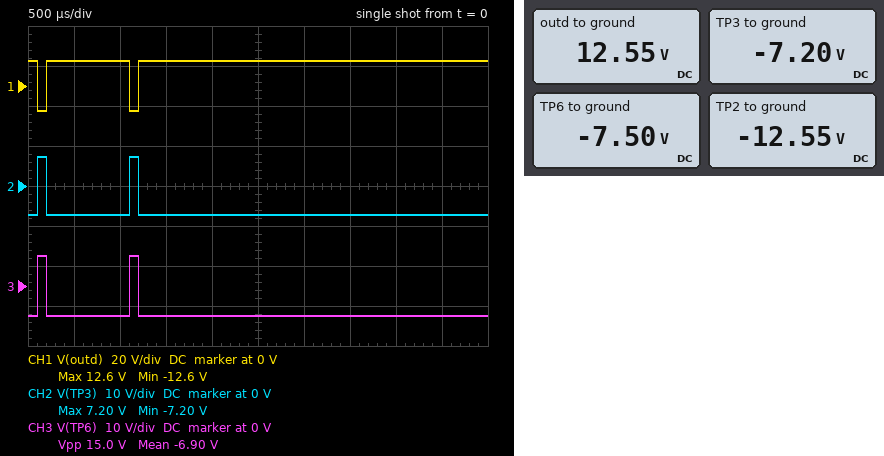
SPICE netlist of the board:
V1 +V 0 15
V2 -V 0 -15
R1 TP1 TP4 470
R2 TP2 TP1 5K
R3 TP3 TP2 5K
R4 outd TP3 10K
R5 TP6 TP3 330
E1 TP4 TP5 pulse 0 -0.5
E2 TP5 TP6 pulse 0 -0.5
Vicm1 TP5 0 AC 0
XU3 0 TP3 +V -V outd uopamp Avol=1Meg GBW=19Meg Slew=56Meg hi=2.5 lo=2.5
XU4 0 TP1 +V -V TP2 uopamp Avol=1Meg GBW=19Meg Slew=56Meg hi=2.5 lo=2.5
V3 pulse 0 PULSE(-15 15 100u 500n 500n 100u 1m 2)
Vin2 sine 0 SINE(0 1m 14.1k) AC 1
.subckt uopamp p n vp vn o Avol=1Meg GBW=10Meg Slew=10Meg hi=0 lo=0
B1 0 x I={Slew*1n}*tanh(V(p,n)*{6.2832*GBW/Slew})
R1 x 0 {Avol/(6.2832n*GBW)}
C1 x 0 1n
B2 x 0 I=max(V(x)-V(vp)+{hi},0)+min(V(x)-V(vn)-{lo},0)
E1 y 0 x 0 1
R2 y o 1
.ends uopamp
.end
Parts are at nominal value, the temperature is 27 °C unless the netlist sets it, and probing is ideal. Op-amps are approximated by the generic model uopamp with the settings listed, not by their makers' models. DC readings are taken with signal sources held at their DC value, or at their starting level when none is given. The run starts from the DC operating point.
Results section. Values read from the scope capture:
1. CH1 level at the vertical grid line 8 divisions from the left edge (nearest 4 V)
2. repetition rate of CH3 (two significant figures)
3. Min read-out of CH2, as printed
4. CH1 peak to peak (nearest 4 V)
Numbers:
12 V
1.0 kHz
-7.20 V
24 V
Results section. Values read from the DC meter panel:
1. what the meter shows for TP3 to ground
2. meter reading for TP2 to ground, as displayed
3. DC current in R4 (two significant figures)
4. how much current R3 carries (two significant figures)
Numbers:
-7.20 V
-12.55 V
2.0 mA
1.1 mA
